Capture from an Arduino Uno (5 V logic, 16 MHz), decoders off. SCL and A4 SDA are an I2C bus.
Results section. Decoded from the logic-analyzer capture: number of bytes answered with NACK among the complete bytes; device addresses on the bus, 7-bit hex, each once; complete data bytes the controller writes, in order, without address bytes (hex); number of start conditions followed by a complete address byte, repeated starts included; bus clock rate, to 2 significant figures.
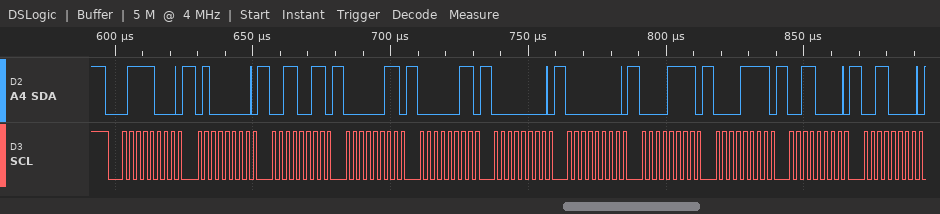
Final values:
0
0x3C
40 33 03 03 00 00 0F 0F 30 30
1
400 kHz
